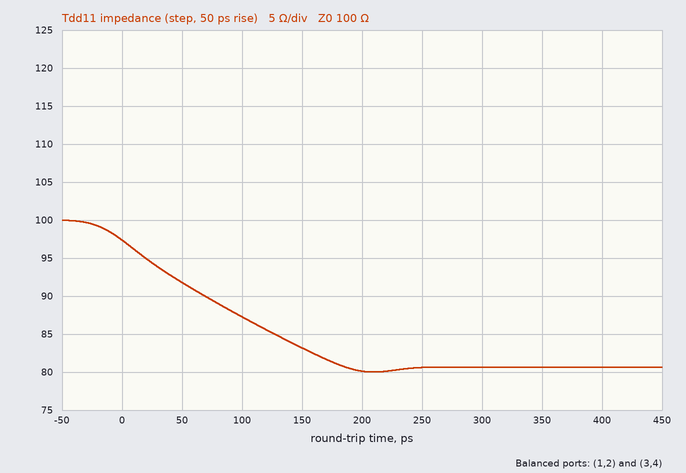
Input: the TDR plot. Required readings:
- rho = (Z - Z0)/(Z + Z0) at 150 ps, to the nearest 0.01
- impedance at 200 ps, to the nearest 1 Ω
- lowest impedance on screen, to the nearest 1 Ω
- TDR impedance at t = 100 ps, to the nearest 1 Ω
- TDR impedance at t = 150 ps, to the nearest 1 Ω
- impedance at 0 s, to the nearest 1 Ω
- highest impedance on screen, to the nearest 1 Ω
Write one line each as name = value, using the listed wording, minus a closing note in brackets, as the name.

rho = (Z - Z0)/(Z + Z0) at 150 ps, to the nearest 0.01 = -0.09
impedance at 200 ps, to the nearest 1 Ω = 80 Ω
lowest impedance on screen, to the nearest 1 Ω = 80 Ω
TDR impedance at t = 100 ps, to the nearest 1 Ω = 87 Ω
TDR impedance at t = 150 ps, to the nearest 1 Ω = 83 Ω
impedance at 0 s, to the nearest 1 Ω = 97 Ω
highest impedance on screen, to the nearest 1 Ω = 100 Ω
